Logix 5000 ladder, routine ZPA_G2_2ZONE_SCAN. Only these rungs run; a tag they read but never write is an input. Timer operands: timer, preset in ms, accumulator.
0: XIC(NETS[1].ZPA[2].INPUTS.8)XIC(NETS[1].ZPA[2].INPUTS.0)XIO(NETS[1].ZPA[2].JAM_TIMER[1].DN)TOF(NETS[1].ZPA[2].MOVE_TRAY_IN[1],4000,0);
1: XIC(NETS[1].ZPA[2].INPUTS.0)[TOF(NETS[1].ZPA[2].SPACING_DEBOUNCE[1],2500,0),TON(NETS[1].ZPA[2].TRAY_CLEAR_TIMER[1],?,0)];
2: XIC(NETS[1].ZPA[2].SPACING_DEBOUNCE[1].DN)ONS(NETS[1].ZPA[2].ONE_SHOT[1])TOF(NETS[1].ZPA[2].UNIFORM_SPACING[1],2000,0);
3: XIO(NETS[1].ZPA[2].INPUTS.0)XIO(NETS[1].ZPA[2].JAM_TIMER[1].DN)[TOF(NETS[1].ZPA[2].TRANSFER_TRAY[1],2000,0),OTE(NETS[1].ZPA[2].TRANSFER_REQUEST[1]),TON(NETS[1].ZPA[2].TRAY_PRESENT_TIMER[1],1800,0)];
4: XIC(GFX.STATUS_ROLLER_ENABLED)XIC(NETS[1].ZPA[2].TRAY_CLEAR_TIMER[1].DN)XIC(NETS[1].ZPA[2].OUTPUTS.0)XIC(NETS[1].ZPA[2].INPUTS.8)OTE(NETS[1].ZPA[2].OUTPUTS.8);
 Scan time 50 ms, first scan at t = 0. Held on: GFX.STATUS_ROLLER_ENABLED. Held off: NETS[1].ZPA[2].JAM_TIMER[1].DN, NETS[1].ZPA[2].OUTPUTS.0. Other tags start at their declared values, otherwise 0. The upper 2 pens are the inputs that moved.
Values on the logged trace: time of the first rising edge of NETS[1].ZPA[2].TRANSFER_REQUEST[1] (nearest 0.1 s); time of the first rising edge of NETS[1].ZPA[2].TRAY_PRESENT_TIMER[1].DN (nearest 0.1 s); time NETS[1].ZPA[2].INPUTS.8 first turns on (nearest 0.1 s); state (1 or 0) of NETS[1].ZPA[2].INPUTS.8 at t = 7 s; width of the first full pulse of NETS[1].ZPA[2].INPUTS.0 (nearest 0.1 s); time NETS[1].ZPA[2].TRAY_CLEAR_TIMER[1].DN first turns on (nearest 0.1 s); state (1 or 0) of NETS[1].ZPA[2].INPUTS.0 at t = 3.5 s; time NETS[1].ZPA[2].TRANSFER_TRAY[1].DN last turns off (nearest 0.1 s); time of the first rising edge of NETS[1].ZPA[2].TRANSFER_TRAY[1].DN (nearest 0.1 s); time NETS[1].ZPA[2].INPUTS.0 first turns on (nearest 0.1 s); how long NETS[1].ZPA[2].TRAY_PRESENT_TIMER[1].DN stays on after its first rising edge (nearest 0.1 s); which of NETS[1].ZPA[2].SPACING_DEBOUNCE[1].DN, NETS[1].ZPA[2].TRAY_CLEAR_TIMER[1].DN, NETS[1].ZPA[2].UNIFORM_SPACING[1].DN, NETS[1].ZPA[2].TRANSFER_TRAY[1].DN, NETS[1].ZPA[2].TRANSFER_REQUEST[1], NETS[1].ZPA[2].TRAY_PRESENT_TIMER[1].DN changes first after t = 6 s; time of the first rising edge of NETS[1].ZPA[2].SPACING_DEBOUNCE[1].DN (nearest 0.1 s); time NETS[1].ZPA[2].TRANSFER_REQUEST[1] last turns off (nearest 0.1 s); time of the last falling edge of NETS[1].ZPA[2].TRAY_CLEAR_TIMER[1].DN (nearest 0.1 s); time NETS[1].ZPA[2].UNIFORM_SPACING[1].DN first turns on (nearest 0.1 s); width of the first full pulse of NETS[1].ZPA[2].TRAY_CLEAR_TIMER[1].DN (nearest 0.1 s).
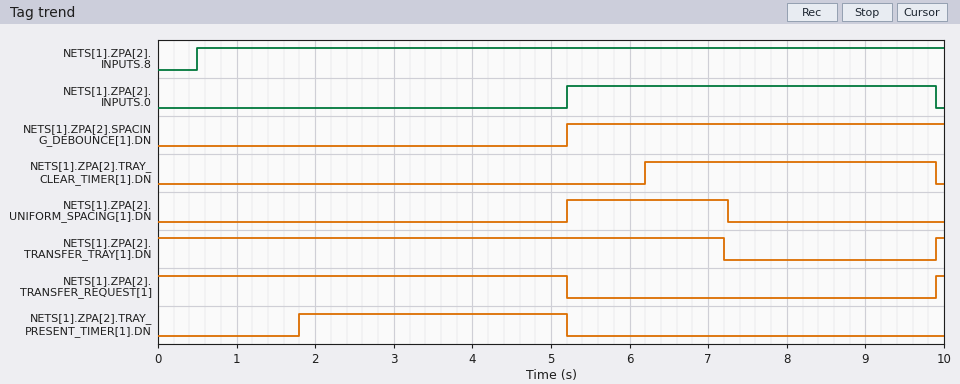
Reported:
9.9 s
1.8 s
0.5 s
1
4.7 s
6.2 s
0
7.2 s
9.9 s
5.2 s
3.4 s
NETS[1].ZPA[2].TRAY_CLEAR_TIMER[1].DN
5.2 s
5.2 s
9.9 s
5.2 s
3.7 s
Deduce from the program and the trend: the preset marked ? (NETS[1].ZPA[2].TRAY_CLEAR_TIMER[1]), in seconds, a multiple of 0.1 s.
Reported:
1.0 s
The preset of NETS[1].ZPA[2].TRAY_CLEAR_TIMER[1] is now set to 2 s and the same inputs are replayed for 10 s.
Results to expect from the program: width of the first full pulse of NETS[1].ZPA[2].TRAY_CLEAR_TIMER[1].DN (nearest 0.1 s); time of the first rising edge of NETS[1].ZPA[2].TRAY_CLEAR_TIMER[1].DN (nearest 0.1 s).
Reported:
2.7 s
7.2 s
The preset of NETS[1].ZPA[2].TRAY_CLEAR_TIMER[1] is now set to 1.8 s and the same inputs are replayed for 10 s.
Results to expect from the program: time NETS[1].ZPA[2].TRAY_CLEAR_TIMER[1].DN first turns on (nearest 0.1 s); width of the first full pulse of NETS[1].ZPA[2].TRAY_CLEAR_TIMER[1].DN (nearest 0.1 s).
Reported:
7.0 s
2.9 s
